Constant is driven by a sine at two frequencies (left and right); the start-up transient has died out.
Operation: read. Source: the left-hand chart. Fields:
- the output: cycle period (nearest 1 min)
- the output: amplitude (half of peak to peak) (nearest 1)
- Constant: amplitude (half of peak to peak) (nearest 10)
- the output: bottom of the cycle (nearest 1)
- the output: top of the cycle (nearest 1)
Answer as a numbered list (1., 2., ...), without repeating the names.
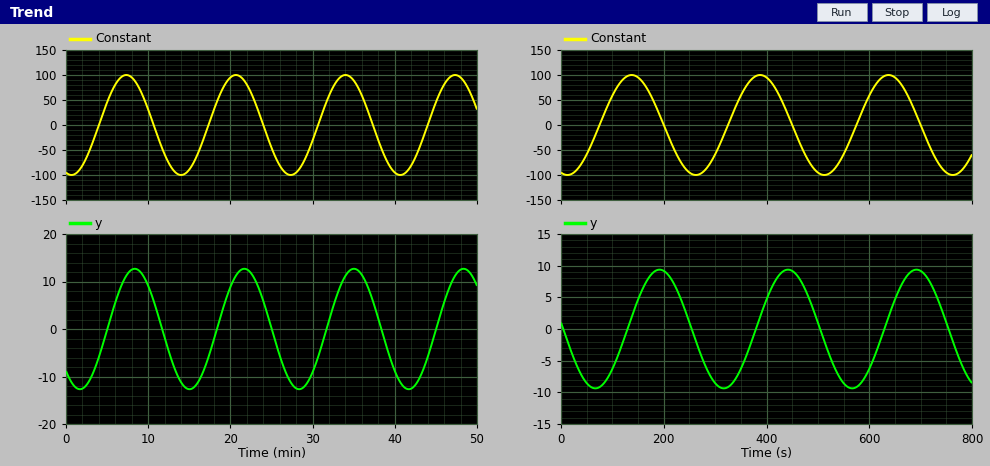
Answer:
1. 13 min
2. 13
3. 100
4. -13
5. 13
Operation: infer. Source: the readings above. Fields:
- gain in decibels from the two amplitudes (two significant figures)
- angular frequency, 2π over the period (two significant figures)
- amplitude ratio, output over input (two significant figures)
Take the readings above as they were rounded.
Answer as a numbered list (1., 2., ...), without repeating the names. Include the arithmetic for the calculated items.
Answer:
1. 20 log10(13 / 100) = -18 dB
2. 2π / 13 = 0.48 rad/min
3. 13 / 100 = 0.13
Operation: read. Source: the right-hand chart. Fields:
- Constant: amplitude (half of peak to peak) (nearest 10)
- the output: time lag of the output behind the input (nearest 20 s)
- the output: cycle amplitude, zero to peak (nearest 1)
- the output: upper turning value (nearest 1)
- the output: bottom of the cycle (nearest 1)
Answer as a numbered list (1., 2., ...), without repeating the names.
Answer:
1. 100
2. 60 s
3. 9
4. 9
5. -9
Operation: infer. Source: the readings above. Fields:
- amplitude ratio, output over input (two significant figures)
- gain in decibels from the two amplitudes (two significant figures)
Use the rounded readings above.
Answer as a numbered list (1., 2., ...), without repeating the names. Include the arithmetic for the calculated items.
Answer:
1. 9 / 100 = 0.090
2. 20 log10(9 / 100) = -21 dB
